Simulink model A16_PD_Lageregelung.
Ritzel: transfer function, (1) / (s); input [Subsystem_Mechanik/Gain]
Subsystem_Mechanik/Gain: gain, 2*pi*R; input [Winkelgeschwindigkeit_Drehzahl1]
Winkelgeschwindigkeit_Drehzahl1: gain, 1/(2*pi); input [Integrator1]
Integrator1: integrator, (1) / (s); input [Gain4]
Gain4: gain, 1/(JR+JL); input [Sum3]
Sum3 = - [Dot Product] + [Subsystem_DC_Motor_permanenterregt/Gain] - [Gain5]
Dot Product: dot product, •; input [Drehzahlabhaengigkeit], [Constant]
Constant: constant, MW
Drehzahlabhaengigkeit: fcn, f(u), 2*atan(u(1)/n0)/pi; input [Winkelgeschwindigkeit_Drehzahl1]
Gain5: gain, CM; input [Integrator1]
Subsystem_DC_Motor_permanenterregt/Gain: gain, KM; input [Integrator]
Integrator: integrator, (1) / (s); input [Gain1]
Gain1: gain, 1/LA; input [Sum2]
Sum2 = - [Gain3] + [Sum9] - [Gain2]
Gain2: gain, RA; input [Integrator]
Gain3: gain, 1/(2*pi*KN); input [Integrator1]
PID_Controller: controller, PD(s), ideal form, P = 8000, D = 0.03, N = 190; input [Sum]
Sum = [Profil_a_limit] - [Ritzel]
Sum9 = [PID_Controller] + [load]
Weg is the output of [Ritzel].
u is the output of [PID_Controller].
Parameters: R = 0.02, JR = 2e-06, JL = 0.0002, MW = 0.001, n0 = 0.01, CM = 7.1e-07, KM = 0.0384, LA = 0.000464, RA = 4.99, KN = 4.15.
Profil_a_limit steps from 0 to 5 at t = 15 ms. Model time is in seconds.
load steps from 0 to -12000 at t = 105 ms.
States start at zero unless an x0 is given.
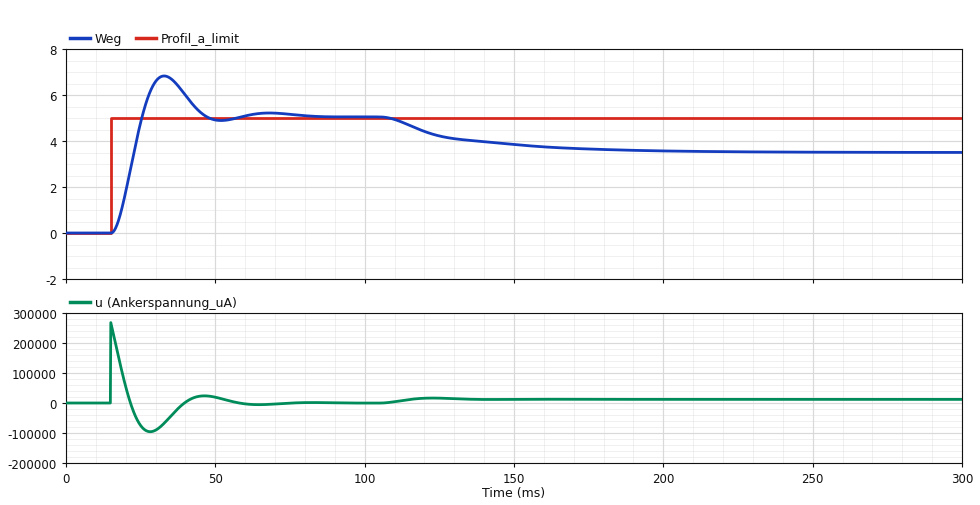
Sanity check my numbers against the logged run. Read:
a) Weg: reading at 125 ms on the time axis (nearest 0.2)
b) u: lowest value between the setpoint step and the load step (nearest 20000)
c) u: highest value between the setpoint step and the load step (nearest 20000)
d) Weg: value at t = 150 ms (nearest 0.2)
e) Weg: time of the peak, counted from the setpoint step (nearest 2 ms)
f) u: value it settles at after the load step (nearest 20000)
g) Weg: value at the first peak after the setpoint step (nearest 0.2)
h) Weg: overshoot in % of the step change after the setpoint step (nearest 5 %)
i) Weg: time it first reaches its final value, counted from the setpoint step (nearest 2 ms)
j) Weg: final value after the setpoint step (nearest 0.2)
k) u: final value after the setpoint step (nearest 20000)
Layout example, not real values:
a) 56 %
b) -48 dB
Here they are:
a) 4.2
b) -100000
c) 260000
d) 3.8
e) 18 ms
f) 20000
g) 6.8
h) 35 %
i) 10 ms
j) 5.0
k) 0
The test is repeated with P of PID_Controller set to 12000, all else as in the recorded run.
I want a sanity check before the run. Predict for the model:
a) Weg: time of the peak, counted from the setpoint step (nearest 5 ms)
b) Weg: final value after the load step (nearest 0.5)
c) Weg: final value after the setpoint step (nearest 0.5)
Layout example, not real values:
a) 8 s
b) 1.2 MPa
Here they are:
a) 15 ms
b) 4.0
c) 5.0
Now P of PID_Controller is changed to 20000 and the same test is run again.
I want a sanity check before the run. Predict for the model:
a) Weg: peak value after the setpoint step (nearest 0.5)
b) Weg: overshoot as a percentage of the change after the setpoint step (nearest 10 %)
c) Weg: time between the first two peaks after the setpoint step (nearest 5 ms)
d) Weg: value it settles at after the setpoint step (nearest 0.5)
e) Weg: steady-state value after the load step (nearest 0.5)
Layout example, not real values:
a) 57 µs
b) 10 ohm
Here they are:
a) 7.5
b) 50 %
c) 20 ms
d) 5.0
e) 4.5
